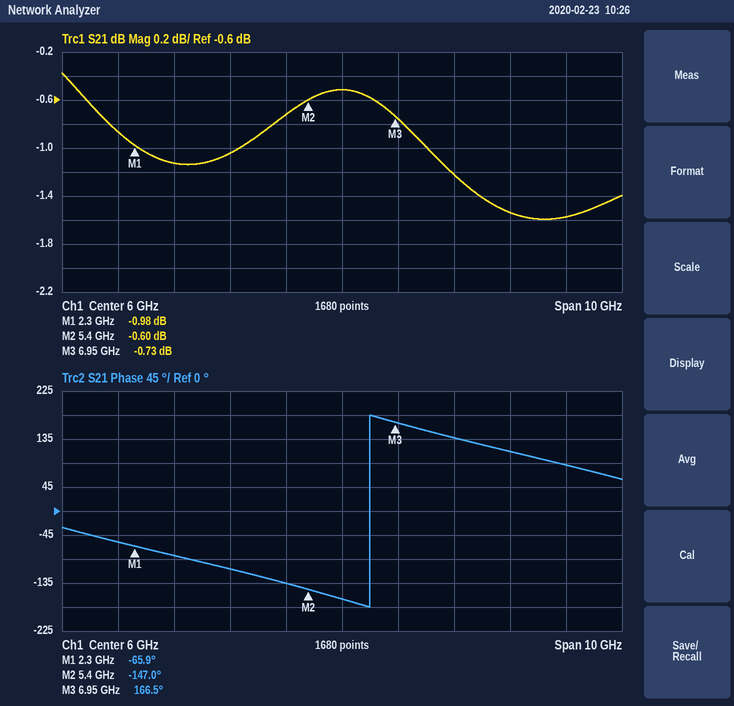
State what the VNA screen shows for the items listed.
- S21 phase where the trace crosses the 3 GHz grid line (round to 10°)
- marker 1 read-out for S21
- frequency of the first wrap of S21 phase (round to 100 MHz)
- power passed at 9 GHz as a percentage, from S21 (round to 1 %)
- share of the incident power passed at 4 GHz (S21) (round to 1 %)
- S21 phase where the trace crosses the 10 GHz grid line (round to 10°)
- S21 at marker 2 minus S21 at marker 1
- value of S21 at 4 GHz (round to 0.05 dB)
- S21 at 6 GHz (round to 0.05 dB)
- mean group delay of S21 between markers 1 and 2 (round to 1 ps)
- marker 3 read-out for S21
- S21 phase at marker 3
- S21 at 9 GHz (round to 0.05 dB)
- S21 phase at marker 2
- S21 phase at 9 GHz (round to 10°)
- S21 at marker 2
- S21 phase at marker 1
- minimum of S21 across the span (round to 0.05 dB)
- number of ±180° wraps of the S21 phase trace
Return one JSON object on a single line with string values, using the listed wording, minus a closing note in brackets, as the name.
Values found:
{"S21 phase where the trace crosses the 3 GHz grid line": "-80°", "marker 1 read-out for S21": "-0.98 dB", "frequency of the first wrap of S21 phase": "6.5 GHz", "power passed at 9 GHz as a percentage, from S21": "70 %", "share of the incident power passed at 4 GHz (S21)": "79 %", "S21 phase where the trace crosses the 10 GHz grid line": "90°", "S21 at marker 2 minus S21 at marker 1": "0.38 dB", "value of S21 at 4 GHz": "-1.05 dB", "S21 at 6 GHz": "-0.50 dB", "mean group delay of S21 between markers 1 and 2": "73 ps", "marker 3 read-out for S21": "-0.73 dB", "S21 phase at marker 3": "166.5°", "S21 at 9 GHz": "-1.55 dB", "S21 phase at marker 2": "-147.0°", "S21 phase at 9 GHz": "110°", "S21 at marker 2": "-0.60 dB", "S21 phase at marker 1": "-65.9°", "minimum of S21 across the span": "-1.60 dB", "number of ±180° wraps of the S21 phase trace": "1"}
